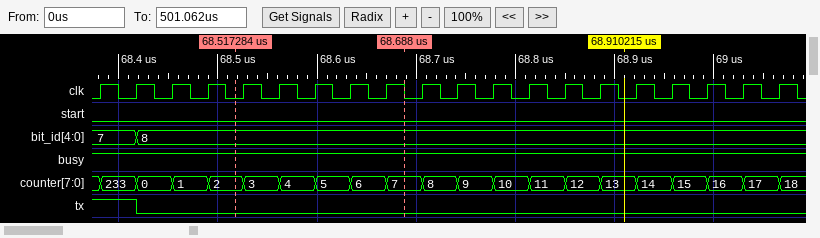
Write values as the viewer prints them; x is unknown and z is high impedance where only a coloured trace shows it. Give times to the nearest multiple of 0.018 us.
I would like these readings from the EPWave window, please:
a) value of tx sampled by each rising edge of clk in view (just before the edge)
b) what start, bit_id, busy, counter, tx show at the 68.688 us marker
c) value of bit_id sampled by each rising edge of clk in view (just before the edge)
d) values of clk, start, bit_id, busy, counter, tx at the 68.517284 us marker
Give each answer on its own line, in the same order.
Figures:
1 1 0 0 0 0 0 0 0 0 0 0 0 0 0 0 0 0 0 0
start=0, bit_id=8, busy=1, counter=7, tx=0
7, 7, 8, 8, 8, 8, 8, 8, 8, 8, 8, 8, 8, 8, 8, 8, 8, 8, 8, 8
clk=0, start=0, bit_id=8, busy=1, counter=2, tx=0
